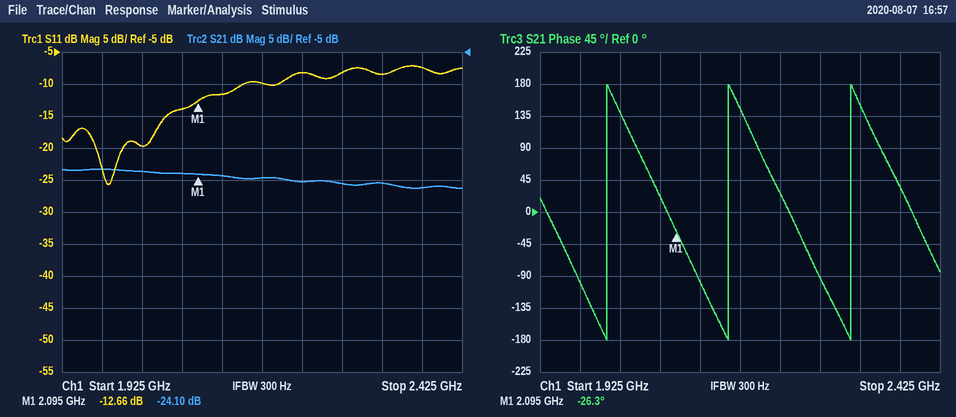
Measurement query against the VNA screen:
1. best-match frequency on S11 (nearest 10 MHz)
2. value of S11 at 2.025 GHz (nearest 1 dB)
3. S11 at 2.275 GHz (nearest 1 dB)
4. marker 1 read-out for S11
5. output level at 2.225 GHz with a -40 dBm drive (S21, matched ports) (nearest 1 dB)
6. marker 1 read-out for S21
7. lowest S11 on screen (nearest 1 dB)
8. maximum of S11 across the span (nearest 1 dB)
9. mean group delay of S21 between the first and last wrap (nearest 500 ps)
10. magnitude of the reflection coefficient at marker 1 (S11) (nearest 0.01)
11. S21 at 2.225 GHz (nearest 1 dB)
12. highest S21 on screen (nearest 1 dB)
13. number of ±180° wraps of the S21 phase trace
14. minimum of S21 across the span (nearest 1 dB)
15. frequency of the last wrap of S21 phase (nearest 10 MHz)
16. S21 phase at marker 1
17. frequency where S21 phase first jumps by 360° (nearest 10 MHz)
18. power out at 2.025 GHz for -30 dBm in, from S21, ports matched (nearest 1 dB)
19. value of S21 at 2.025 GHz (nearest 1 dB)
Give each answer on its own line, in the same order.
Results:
1.98 GHz
-20 dB
-8 dB
-12.66 dB
-65 dBm
-24.10 dB
-26 dB
-7 dB
6.5 ns
0.23
-25 dB
-23 dB
3
-26 dB
2.31 GHz
-26.3°
2.01 GHz
-54 dBm
-24 dB
